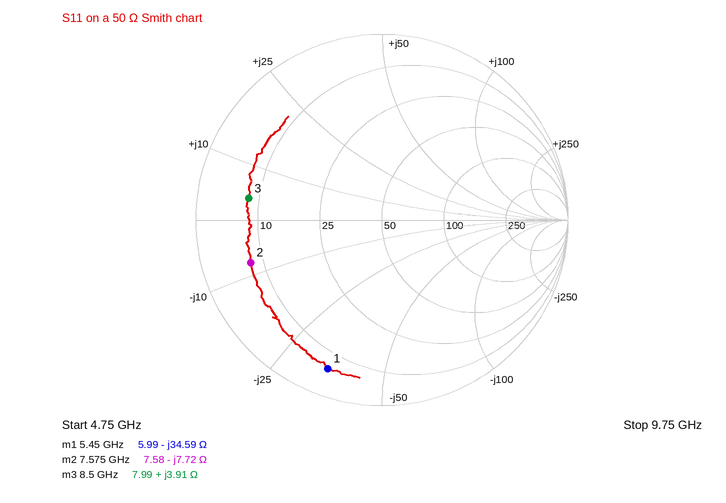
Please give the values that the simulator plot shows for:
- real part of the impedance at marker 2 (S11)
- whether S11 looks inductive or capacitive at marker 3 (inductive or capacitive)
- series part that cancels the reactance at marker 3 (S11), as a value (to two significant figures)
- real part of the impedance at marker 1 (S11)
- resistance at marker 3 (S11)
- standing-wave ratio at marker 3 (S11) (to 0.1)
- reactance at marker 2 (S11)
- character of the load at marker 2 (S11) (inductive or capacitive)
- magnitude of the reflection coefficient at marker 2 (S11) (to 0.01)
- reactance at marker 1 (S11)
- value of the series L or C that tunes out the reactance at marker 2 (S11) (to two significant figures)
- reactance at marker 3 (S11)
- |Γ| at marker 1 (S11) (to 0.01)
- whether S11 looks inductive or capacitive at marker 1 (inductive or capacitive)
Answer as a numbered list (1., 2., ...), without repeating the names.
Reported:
1. 7.58 Ω
2. inductive
3. 4.8 pF
4. 5.99 Ω
5. 7.99 Ω
6. 6.3
7. -7.72 Ω
8. capacitive
9. 0.74
10. -34.59 Ω
11. 160 pH
12. +3.91 Ω
13. 0.85
14. capacitive
